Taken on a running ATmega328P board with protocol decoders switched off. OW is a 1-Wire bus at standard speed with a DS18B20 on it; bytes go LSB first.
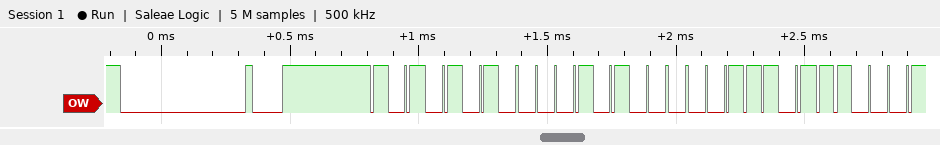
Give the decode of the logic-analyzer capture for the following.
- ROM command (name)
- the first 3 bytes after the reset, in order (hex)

Match ROM
55 28 B8
